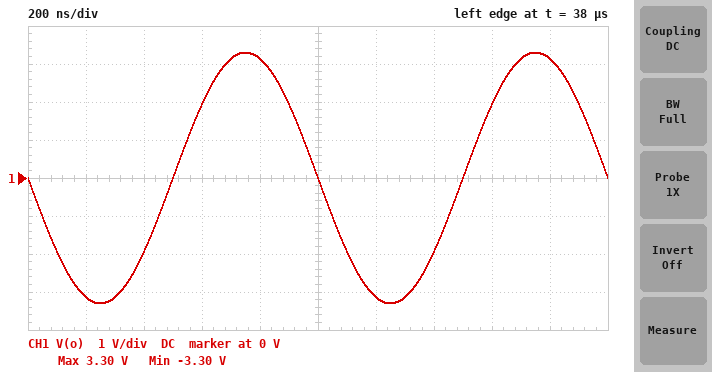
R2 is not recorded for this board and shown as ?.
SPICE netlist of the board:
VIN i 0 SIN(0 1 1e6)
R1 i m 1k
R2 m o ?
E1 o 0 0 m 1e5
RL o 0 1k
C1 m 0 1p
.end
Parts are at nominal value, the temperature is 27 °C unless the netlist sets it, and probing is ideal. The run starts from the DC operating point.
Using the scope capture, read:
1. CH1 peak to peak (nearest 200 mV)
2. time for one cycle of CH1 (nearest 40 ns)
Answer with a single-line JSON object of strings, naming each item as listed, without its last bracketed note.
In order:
{"CH1 peak to peak": "6.6 V", "time for one cycle of CH1": "1.00 µs"}
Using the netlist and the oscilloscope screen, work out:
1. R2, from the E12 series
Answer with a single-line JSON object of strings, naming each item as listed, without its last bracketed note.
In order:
{"R2, from the E12 series": "3.3 kΩ"}
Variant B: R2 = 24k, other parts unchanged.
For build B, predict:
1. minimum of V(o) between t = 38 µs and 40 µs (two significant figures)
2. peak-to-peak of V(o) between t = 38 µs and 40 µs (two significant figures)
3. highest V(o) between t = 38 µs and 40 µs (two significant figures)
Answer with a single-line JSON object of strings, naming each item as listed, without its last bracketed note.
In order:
{"minimum of V(o) between t = 38 µs and 40 µs": "-24 V", "peak-to-peak of V(o) between t = 38 µs and 40 µs": "48 V", "highest V(o) between t = 38 µs and 40 µs": "24 V"}
